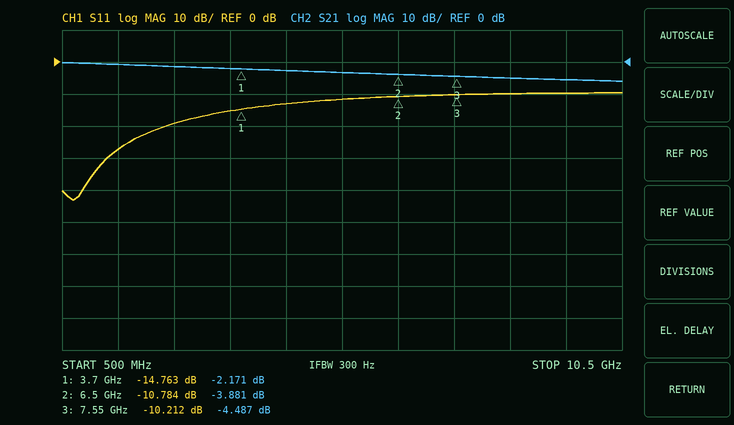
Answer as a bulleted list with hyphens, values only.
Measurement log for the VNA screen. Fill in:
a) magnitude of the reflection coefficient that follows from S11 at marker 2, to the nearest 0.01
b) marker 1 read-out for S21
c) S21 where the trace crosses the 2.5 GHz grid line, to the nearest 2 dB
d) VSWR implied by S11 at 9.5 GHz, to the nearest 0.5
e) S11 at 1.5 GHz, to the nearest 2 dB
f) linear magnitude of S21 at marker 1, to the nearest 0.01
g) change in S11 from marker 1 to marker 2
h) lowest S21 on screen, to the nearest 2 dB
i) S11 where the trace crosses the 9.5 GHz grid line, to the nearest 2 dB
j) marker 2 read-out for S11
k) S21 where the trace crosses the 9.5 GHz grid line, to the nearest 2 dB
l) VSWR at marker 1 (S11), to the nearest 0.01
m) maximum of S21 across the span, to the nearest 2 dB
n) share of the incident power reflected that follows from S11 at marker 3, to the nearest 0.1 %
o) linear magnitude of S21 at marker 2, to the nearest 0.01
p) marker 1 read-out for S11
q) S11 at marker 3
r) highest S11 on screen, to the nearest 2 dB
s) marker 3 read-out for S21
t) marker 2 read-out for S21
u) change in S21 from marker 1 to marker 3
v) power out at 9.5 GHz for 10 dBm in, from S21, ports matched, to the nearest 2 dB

- 0.29
- -2.171 dB
- -2 dB
- 2.0
- -28 dB
- 0.78
- 3.979 dB
- -6 dB
- -10 dB
- -10.784 dB
- -6 dB
- 1.45
- 0 dB
- 9.5 %
- 0.64
- -14.763 dB
- -10.212 dB
- -10 dB
- -4.487 dB
- -3.881 dB
- -2.316 dB
- 4 dBm
